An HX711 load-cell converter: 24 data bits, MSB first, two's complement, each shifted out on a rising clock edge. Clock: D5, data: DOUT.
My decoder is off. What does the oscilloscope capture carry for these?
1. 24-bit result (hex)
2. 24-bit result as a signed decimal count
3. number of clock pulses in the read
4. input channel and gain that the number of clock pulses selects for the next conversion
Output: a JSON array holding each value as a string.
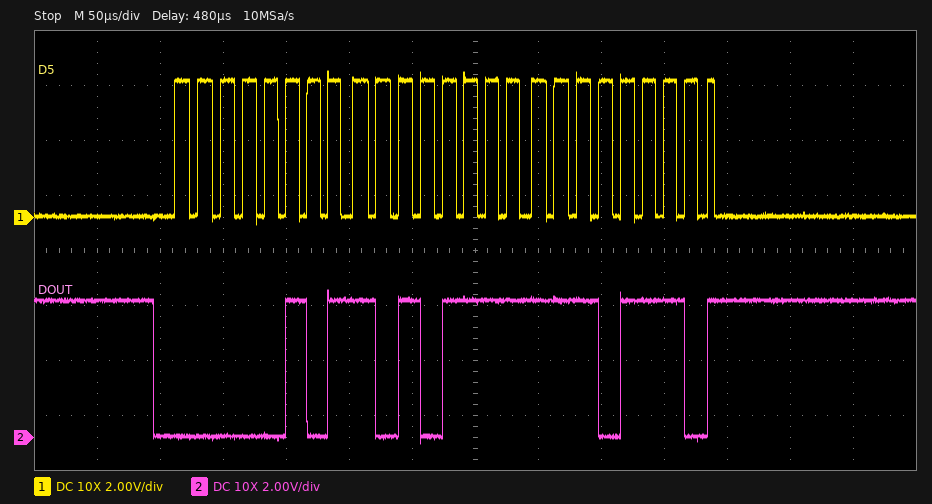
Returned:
["0x05AFEE", "372718", "25", "channel A, gain 128"]
